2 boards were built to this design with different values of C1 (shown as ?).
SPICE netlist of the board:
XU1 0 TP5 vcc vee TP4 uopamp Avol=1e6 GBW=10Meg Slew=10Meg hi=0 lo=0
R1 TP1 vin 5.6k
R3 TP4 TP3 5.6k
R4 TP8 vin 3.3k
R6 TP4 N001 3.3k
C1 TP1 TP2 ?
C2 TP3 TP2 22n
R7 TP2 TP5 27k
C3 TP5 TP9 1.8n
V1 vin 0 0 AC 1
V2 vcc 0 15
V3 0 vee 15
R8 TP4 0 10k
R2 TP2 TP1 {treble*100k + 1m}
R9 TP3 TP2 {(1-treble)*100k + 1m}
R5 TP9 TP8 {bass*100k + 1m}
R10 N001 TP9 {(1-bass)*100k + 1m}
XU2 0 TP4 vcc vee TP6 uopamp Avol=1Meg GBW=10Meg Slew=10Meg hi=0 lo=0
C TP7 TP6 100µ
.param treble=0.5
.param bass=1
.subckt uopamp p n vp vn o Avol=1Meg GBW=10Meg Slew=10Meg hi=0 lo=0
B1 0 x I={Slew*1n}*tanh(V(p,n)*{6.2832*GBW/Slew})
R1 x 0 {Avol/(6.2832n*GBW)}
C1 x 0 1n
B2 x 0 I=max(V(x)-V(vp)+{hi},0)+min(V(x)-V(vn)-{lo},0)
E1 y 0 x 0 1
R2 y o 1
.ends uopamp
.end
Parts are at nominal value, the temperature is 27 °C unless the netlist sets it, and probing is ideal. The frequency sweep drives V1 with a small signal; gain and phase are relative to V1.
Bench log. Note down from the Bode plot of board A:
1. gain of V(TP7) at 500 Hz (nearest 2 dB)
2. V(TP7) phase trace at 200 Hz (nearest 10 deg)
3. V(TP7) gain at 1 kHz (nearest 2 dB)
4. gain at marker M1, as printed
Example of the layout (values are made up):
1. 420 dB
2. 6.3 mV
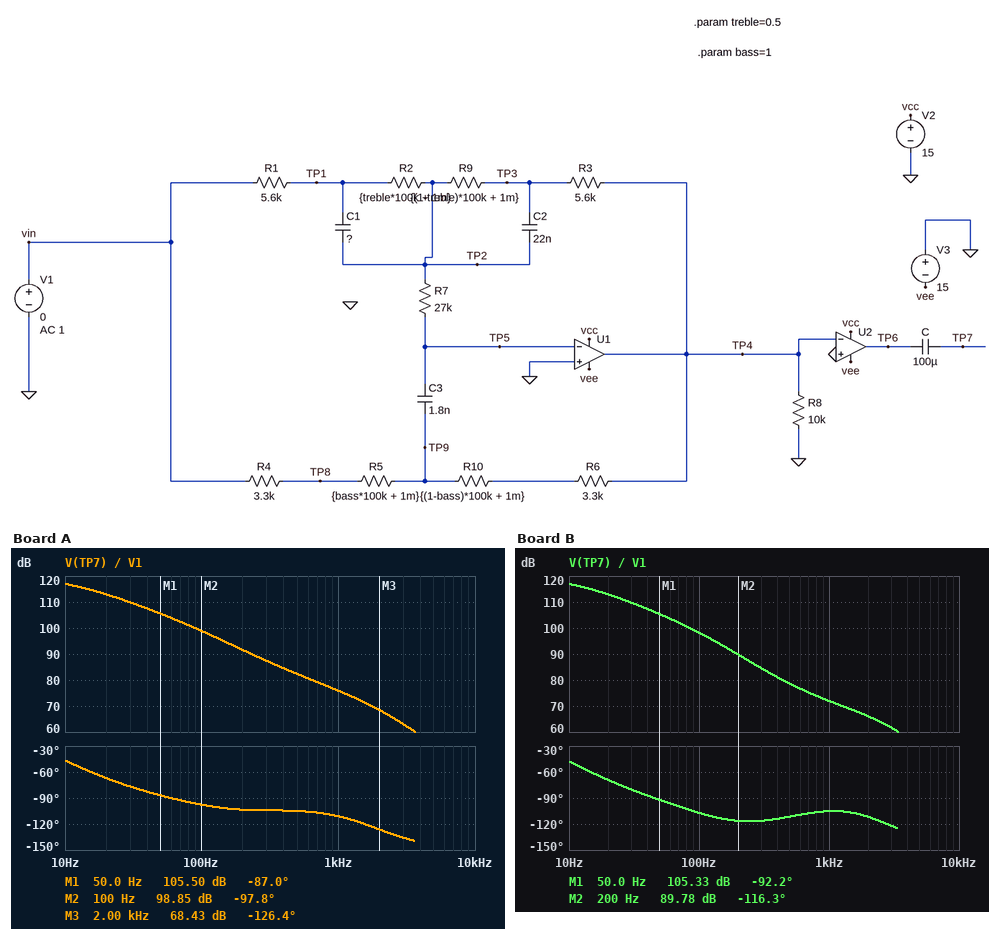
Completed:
1. 82 dB
2. -100 deg
3. 76 dB
4. 105.50 dB
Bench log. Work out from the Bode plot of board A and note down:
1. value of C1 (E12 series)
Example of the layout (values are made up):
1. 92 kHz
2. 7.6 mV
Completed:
1. 15 nF
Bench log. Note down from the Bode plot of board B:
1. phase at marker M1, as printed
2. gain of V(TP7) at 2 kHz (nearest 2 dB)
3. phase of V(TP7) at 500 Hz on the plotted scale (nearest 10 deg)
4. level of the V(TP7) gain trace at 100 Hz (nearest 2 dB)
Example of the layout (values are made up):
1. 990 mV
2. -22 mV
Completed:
1. -92.2 deg
2. 66 dB
3. -110 deg
4. 98 dB
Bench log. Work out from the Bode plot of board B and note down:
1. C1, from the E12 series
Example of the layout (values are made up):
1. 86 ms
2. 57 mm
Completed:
1. 8.2 nF
